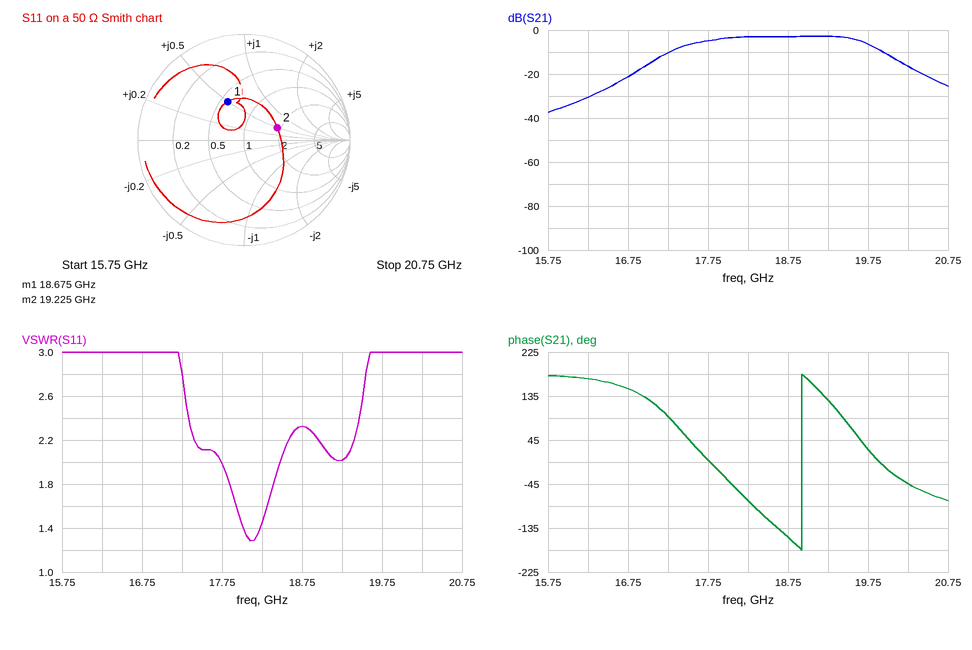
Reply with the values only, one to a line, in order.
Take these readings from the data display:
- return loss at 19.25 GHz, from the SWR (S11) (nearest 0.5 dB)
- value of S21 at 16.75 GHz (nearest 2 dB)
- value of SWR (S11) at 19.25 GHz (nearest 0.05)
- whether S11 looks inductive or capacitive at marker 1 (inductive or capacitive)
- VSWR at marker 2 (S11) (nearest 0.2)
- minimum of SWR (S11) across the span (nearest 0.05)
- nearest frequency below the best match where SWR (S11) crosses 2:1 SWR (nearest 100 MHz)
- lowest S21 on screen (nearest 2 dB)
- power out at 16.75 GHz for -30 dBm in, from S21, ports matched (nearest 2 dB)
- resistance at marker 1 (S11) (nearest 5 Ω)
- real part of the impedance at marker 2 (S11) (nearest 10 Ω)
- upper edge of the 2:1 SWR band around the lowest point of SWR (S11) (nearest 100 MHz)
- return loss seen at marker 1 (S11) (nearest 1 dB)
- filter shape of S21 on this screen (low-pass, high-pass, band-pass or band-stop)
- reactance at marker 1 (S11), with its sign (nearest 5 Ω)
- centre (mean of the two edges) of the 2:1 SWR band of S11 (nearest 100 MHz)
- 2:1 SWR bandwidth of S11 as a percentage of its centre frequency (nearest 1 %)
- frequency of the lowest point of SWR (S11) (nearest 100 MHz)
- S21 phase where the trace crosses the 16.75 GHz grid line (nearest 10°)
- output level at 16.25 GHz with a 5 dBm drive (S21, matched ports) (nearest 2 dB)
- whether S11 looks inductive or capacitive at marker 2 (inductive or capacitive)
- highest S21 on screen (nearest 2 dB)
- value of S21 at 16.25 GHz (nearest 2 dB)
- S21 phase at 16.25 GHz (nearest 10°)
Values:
9.5 dB
-22 dB
2.00
inductive
2.0
1.30
17.7 GHz
-38 dB
-52 dBm
30 Ω
90 Ω
18.5 GHz
8 dB
band-pass
+25 Ω
18.1 GHz
4 %
18.1 GHz
150°
-26 dBm
inductive
-2 dB
-30 dB
170°
